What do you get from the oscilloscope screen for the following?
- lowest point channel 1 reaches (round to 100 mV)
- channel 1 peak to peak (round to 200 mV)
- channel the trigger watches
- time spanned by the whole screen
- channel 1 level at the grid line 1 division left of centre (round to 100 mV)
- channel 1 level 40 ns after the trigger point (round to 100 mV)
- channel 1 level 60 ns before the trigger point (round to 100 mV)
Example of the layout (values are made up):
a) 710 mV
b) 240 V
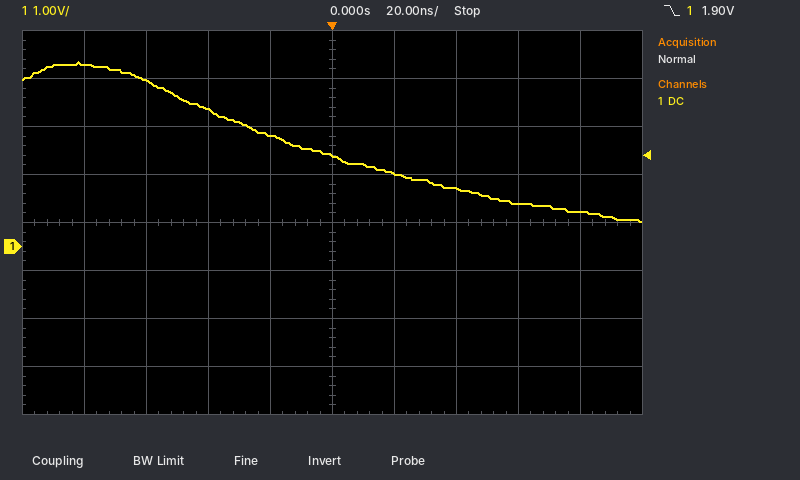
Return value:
a) 500 mV
b) 3.4 V
c) channel 1
d) 200 ns
e) 2.3 V
f) 1.2 V
g) 3.5 V
